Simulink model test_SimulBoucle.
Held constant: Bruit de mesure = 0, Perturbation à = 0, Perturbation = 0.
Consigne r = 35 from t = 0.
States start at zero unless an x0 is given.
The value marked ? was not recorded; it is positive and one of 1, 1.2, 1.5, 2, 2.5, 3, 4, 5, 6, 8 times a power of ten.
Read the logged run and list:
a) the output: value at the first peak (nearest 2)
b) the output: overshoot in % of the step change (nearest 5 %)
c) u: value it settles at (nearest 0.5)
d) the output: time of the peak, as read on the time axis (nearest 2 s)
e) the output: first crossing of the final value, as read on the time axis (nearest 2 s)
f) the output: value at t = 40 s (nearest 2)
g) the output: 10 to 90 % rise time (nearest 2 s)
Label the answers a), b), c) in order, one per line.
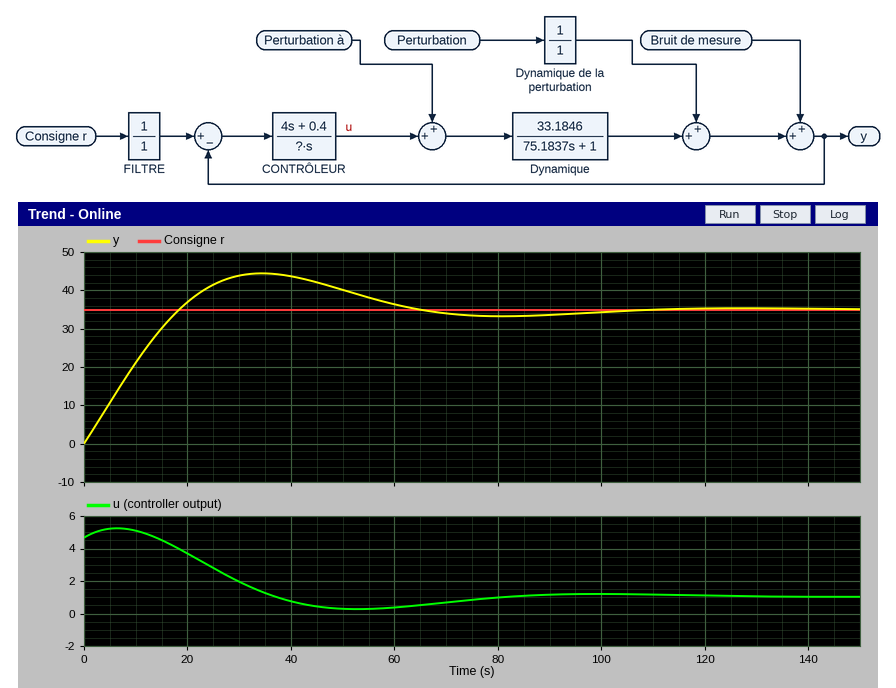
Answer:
a) 44
b) 25 %
c) 1.0
d) 34 s
e) 18 s
f) 44
g) 14 s
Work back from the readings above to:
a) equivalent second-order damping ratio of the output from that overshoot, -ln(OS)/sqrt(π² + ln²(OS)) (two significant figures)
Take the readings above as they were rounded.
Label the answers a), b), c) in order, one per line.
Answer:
a) 0.40
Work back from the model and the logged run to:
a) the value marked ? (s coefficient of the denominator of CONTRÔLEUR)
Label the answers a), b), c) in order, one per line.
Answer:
a) 30
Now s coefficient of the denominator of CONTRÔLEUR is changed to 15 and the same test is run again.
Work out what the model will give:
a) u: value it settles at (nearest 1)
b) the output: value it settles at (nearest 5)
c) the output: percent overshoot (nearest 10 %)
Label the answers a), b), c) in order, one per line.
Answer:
a) 1
b) 35
c) 20 %
